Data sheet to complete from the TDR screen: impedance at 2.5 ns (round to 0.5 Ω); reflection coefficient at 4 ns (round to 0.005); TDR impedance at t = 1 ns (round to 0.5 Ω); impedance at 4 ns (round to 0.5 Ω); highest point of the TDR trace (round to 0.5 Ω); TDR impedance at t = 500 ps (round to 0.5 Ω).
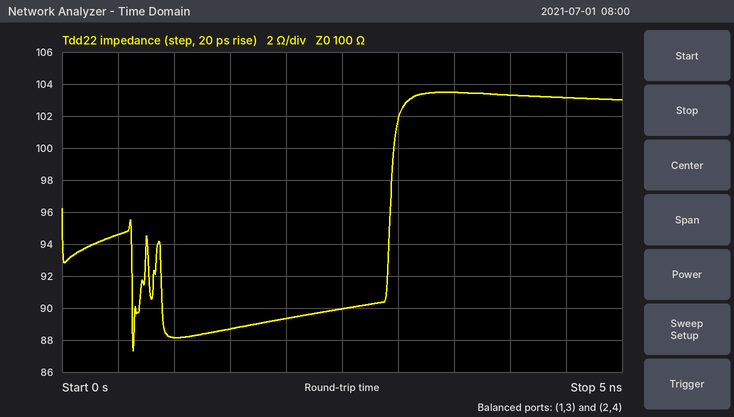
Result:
90.0 Ω
+0.015
88.0 Ω
103.5 Ω
103.5 Ω
94.5 Ω
